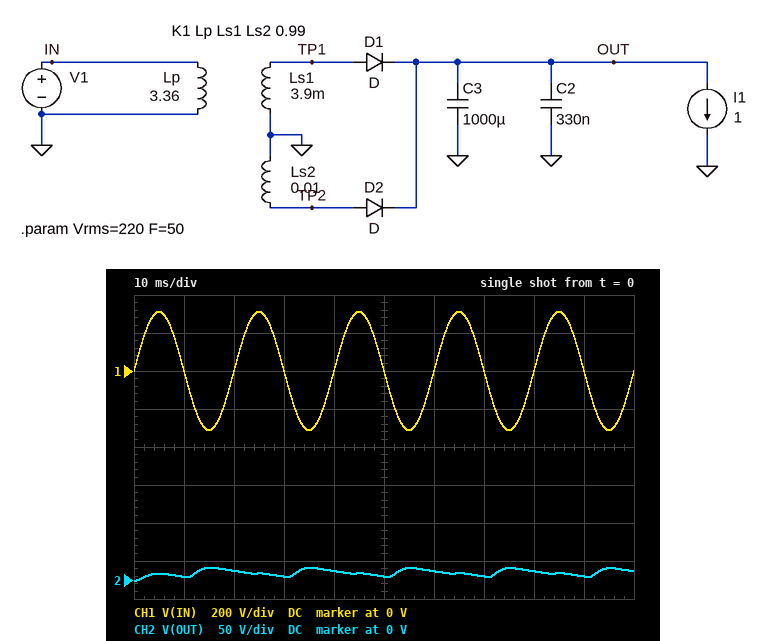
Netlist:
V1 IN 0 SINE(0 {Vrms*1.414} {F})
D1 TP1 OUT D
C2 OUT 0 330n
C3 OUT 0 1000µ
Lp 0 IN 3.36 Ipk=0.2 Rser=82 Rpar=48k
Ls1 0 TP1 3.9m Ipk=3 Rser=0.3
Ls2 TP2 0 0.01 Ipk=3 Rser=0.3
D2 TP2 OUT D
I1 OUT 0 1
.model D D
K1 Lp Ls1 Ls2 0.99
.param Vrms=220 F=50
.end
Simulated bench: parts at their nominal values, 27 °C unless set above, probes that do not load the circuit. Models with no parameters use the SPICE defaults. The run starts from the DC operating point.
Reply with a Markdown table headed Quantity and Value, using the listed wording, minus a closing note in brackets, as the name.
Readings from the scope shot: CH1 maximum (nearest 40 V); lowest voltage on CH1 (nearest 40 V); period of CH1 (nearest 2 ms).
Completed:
| Quantity | Value |
|---|---|
| CH1 maximum | 320 V |
| lowest voltage on CH1 | -320 V |
| period of CH1 | 20 ms |
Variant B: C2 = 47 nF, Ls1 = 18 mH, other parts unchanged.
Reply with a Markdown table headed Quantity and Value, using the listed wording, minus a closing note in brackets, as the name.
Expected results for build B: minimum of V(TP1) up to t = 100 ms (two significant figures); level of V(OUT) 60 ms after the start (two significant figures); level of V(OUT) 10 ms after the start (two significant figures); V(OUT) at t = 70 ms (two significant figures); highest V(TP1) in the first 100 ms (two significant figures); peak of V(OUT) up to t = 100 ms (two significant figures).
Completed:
| Quantity | Value |
|---|---|
| minimum of V(TP1) up to t = 100 ms | -23 V |
| level of V(OUT) 60 ms after the start | 11 V |
| level of V(OUT) 10 ms after the start | 16 V |
| V(OUT) at t = 70 ms | 17 V |
| highest V(TP1) in the first 100 ms | 22 V |
| peak of V(OUT) up to t = 100 ms | 21 V |
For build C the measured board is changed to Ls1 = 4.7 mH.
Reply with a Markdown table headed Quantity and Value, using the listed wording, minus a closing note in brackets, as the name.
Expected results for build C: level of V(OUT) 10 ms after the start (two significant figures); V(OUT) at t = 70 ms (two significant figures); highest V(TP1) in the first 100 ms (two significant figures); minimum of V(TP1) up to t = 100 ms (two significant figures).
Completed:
| Quantity | Value |
|---|---|
| level of V(OUT) 10 ms after the start | 5.1 V |
| V(OUT) at t = 70 ms | 5.6 V |
| highest V(TP1) in the first 100 ms | 11 V |
| minimum of V(TP1) up to t = 100 ms | -12 V |
